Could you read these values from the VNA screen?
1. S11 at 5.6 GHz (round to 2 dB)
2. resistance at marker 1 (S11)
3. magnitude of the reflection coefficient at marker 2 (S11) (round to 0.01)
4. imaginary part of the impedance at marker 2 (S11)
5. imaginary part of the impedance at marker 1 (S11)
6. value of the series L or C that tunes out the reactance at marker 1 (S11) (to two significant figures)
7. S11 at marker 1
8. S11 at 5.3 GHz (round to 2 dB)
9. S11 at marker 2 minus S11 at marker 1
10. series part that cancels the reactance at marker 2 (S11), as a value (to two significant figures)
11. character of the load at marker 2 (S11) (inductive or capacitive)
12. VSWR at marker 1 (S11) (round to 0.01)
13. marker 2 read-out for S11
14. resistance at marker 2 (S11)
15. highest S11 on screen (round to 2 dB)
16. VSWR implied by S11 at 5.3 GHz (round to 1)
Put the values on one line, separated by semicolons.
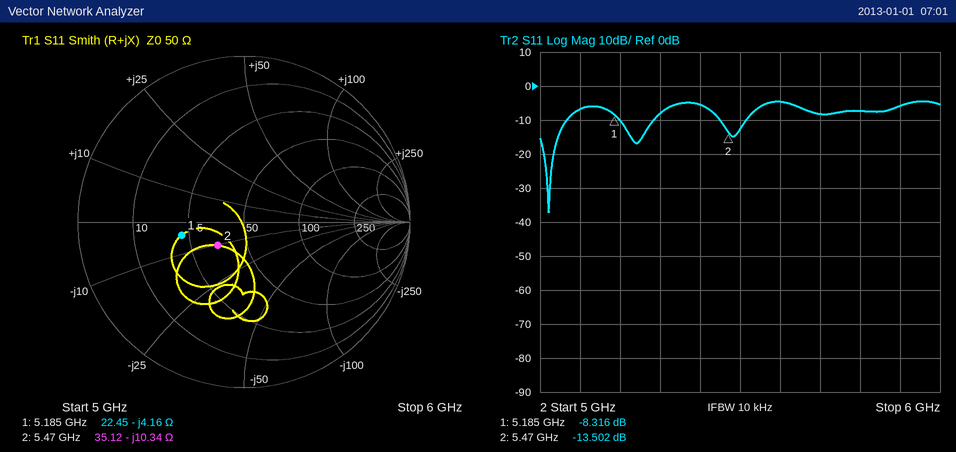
-4 dB; 22.45 Ω; 0.21; -10.34 Ω; -4.16 Ω; 130 pH; -8.316 dB; -8 dB; -5.186 dB; 300 pH; capacitive; 2.25; -13.502 dB; 35.12 Ω; -4 dB; 2
